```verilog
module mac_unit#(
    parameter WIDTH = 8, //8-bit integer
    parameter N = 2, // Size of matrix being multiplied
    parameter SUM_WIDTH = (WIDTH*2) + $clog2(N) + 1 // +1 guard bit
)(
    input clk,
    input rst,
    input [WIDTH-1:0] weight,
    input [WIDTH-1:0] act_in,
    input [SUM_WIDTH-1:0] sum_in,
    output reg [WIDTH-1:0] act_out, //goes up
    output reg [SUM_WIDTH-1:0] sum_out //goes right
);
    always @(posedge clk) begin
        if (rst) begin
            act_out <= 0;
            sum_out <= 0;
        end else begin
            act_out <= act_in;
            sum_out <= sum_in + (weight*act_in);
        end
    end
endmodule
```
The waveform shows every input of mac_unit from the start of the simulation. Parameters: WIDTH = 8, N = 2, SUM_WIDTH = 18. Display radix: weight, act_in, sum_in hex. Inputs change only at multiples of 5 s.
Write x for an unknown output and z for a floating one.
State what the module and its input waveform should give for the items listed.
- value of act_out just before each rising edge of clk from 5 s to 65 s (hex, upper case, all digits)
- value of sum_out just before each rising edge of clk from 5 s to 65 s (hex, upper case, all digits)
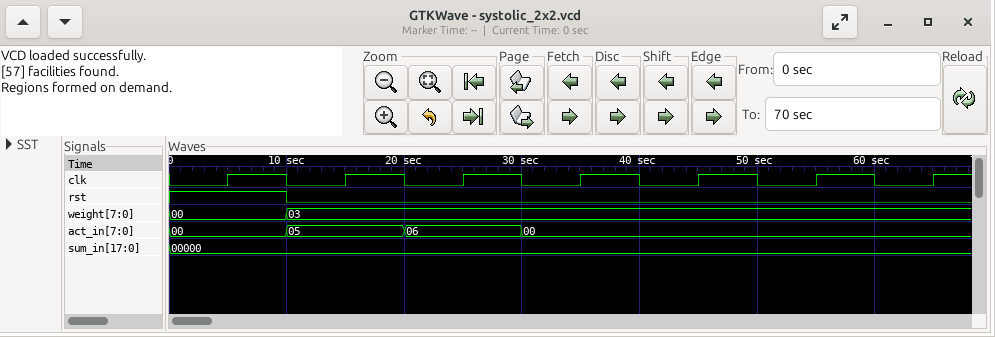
x, 00, 05, 06, 00, 00, 00
x, 00000, 0000F, 00012, 00000, 00000, 00000
